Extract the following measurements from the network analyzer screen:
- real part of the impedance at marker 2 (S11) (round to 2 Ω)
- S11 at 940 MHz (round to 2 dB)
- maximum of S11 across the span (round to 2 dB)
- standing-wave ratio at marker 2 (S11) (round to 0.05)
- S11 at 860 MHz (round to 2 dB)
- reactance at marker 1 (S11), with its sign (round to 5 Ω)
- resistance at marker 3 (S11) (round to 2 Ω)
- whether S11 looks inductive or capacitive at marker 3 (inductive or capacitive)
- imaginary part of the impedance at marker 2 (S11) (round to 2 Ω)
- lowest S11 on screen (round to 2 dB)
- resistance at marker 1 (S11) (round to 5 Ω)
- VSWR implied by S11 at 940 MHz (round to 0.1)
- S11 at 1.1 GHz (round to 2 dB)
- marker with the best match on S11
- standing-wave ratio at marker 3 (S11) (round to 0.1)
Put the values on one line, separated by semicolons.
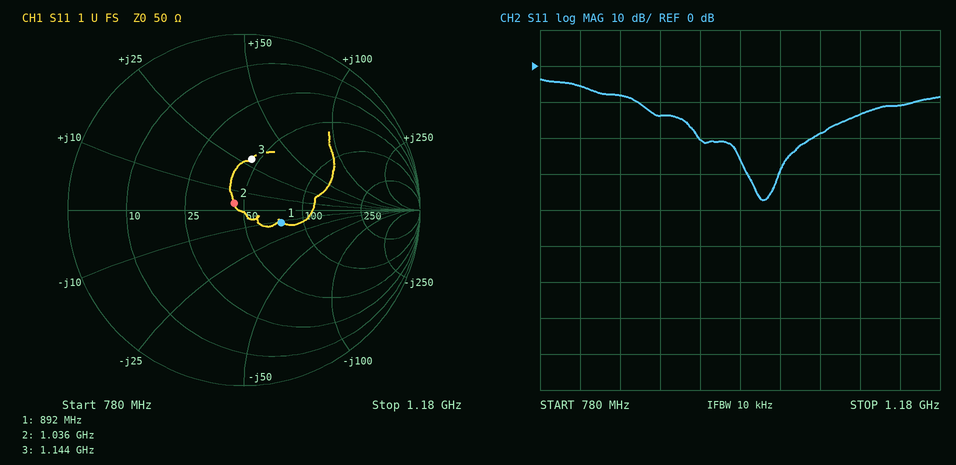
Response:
44 Ω; -20 dB; -4 dB; 1.15; -8 dB; -10 Ω; 46 Ω; inductive; +4 Ω; -38 dB; 75 Ω; 1.2; -14 dB; marker 2; 1.8
